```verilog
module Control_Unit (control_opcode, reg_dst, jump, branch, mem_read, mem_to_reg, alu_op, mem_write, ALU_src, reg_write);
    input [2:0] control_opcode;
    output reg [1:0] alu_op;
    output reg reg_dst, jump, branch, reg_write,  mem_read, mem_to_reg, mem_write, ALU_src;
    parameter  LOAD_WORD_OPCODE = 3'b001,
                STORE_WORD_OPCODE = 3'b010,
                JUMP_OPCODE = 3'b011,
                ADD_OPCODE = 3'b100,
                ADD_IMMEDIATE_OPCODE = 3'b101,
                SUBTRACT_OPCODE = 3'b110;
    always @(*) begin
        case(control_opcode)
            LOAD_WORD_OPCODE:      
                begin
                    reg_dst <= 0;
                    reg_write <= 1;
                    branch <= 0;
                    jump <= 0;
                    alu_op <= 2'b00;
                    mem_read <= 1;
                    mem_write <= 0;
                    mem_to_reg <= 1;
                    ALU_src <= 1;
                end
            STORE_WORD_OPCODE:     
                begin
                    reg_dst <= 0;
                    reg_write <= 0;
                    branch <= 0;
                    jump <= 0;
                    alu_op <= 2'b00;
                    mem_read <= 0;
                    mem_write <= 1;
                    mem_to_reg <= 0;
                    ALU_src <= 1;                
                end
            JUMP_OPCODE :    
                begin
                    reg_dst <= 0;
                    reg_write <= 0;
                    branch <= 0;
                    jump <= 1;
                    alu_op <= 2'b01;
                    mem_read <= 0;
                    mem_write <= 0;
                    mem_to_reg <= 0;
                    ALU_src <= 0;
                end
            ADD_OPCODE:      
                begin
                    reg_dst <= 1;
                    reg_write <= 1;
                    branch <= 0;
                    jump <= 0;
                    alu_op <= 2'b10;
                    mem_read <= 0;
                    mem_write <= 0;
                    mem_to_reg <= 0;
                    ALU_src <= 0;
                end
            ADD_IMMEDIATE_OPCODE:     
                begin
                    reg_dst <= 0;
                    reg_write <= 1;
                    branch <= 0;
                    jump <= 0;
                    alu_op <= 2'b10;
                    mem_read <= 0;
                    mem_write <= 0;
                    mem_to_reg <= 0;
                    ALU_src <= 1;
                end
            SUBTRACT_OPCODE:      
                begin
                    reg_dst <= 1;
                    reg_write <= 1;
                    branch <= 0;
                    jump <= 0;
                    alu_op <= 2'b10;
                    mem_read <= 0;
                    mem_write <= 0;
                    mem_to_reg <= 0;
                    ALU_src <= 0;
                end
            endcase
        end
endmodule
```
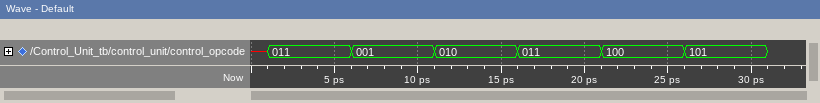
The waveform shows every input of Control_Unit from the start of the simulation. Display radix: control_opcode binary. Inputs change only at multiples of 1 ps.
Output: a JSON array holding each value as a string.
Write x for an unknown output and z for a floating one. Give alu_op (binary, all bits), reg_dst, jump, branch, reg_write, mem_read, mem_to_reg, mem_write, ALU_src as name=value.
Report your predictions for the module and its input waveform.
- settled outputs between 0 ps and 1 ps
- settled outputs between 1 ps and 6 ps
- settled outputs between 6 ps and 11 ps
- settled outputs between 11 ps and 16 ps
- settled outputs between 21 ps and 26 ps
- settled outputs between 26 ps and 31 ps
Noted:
["alu_op=x, reg_dst=x, jump=x, branch=x, reg_write=x, mem_read=x, mem_to_reg=x, mem_write=x, ALU_src=x", "alu_op=01, reg_dst=0, jump=1, branch=0, reg_write=0, mem_read=0, mem_to_reg=0, mem_write=0, ALU_src=0", "alu_op=00, reg_dst=0, jump=0, branch=0, reg_write=1, mem_read=1, mem_to_reg=1, mem_write=0, ALU_src=1", "alu_op=00, reg_dst=0, jump=0, branch=0, reg_write=0, mem_read=0, mem_to_reg=0, mem_write=1, ALU_src=1", "alu_op=10, reg_dst=1, jump=0, branch=0, reg_write=1, mem_read=0, mem_to_reg=0, mem_write=0, ALU_src=0", "alu_op=10, reg_dst=0, jump=0, branch=0, reg_write=1, mem_read=0, mem_to_reg=0, mem_write=0, ALU_src=1"]
